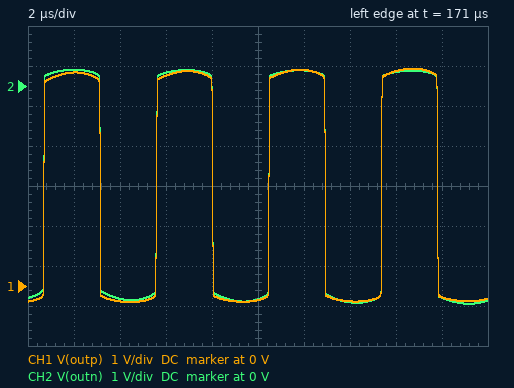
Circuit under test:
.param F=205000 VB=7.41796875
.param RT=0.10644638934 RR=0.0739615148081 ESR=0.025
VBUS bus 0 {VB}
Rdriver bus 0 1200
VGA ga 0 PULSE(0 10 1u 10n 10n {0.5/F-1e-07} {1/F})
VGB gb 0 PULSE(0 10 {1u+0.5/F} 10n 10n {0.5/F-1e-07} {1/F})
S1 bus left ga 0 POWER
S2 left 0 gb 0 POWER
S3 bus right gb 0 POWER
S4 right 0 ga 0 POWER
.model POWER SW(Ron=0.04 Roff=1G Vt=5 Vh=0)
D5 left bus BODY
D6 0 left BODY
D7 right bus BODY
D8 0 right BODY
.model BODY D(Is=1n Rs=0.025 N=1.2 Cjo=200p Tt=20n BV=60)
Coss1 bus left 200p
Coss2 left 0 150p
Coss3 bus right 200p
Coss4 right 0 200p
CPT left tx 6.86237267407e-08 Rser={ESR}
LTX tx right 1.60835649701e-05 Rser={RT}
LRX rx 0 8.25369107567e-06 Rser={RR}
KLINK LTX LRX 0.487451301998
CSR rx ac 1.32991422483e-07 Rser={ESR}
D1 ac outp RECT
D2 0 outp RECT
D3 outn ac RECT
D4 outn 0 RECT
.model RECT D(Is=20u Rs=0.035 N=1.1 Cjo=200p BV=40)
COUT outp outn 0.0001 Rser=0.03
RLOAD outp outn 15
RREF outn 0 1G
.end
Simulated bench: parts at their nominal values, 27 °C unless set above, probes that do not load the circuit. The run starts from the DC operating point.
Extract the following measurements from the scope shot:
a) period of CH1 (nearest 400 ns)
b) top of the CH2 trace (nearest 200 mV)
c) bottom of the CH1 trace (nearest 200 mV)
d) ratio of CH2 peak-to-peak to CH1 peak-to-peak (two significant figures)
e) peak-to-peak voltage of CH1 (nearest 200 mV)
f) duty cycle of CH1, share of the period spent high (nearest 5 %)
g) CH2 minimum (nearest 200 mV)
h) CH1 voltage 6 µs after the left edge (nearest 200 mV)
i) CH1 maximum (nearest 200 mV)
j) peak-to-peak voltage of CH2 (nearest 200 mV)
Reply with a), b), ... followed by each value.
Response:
a) 4.8 µs
b) 400 mV
c) -400 mV
d) 1.0
e) 5.8 V
f) 50 %
g) -5.4 V
h) 5.2 V
i) 5.4 V
j) 5.8 V
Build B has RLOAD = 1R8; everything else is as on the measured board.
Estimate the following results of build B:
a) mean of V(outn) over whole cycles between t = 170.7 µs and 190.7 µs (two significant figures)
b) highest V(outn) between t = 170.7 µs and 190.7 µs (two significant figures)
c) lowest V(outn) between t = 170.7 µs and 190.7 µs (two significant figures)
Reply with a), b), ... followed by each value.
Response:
a) -1.9 V
b) 490 mV
c) -4.3 V
